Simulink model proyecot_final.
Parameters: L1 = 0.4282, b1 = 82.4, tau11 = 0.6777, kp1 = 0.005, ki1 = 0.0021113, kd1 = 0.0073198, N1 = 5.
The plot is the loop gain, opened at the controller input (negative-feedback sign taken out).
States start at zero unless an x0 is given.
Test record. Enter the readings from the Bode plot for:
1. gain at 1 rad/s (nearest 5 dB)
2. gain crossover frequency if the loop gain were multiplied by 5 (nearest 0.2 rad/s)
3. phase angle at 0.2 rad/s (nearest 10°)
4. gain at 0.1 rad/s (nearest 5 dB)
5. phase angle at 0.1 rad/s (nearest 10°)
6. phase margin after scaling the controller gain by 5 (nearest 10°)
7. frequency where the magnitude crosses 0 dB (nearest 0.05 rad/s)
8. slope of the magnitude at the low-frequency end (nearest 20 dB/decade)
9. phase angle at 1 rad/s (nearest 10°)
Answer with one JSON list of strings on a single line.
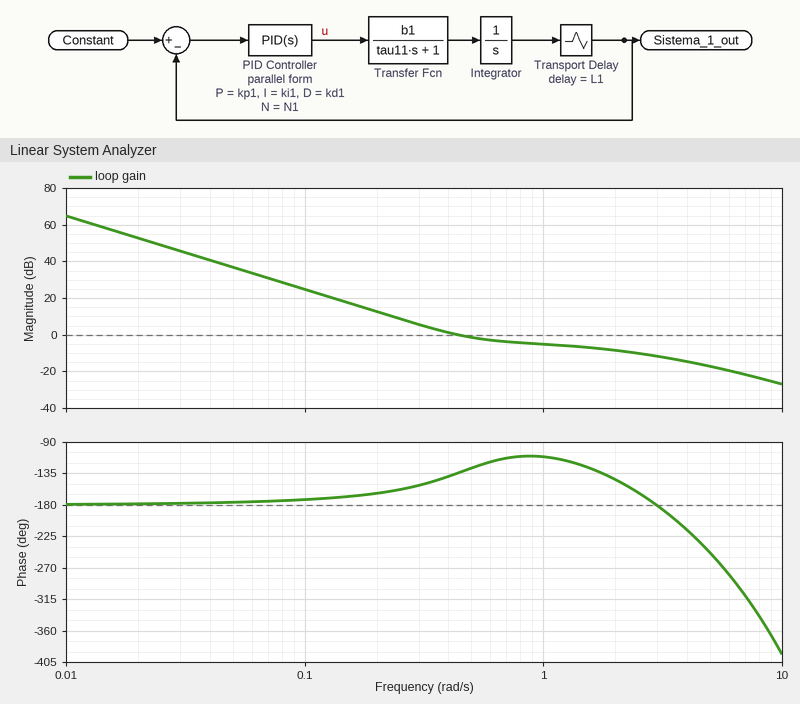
["-5 dB", "3.8 rad/s", "-160°", "25 dB", "-170°", "-30°", "0.45 rad/s", "-40 dB/decade", "-110°"]
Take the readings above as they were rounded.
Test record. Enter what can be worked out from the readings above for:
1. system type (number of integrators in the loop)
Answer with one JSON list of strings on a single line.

["2"]
